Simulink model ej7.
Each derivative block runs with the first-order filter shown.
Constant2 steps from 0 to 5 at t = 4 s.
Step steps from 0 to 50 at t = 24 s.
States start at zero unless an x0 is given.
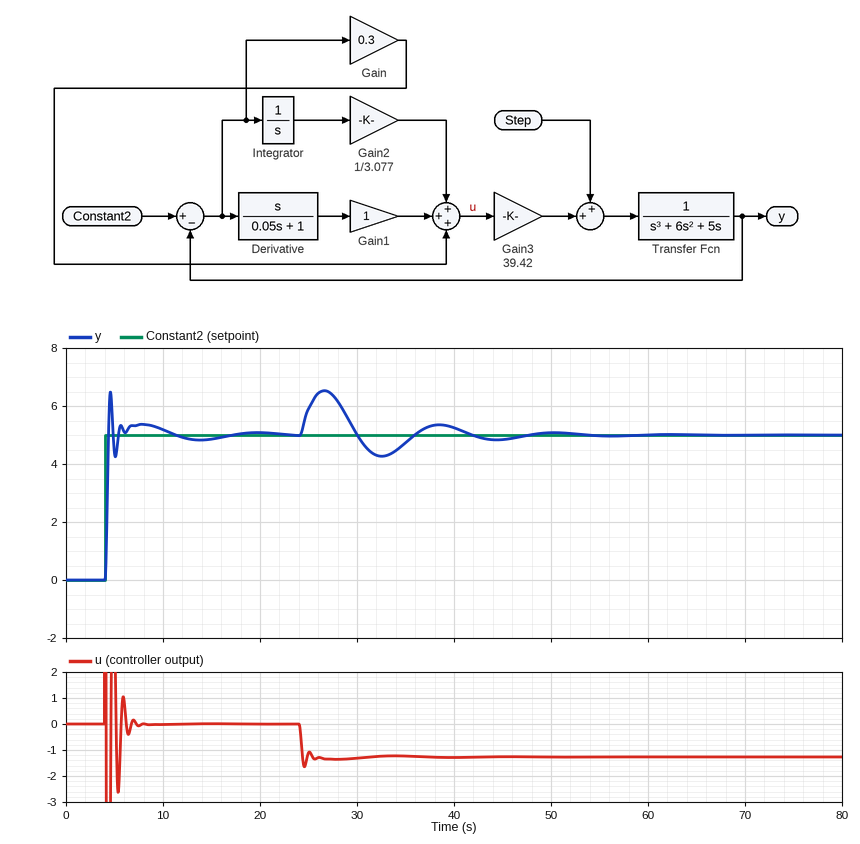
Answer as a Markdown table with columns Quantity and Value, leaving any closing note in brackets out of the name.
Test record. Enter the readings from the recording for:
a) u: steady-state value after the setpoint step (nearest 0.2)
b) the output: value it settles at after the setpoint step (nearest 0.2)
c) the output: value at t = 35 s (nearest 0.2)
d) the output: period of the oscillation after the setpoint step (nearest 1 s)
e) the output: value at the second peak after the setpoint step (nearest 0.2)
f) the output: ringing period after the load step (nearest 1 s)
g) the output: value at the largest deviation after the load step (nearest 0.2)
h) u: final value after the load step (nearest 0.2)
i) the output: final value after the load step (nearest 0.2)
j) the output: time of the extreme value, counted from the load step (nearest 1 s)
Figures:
| Quantity | Value |
|---|---|
| u: steady-state value after the setpoint step | 0.0 |
| the output: value it settles at after the setpoint step | 5.0 |
| the output: value at t = 35 s | 4.8 |
| the output: period of the oscillation after the setpoint step | 3 s |
| the output: value at the second peak after the setpoint step | 5.4 |
| the output: ringing period after the load step | 12 s |
| the output: value at the largest deviation after the load step | 6.6 |
| u: final value after the load step | -1.2 |
| the output: final value after the load step | 5.0 |
| the output: time of the extreme value, counted from the load step | 3 s |
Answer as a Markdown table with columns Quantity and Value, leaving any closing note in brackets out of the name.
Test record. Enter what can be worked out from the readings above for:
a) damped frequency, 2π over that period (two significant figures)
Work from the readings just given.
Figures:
| Quantity | Value |
|---|---|
| damped frequency, 2π over that period | 2.1 rad/s |
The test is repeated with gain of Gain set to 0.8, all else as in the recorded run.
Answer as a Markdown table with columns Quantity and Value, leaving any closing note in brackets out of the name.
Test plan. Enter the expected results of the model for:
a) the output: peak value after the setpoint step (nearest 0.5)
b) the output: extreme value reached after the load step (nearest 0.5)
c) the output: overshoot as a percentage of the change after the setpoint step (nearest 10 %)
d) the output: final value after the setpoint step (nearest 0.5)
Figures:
| Quantity | Value |
|---|---|
| the output: peak value after the setpoint step | 7.0 |
| the output: extreme value reached after the load step | 6.0 |
| the output: overshoot as a percentage of the change after the setpoint step | 40 % |
| the output: final value after the setpoint step | 5.0 |
